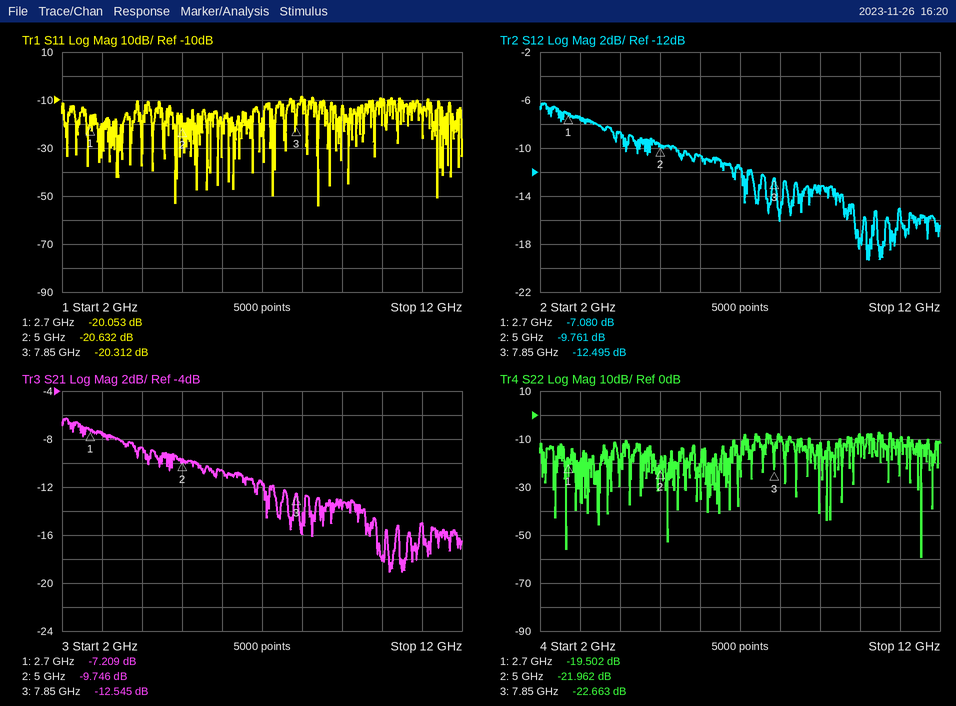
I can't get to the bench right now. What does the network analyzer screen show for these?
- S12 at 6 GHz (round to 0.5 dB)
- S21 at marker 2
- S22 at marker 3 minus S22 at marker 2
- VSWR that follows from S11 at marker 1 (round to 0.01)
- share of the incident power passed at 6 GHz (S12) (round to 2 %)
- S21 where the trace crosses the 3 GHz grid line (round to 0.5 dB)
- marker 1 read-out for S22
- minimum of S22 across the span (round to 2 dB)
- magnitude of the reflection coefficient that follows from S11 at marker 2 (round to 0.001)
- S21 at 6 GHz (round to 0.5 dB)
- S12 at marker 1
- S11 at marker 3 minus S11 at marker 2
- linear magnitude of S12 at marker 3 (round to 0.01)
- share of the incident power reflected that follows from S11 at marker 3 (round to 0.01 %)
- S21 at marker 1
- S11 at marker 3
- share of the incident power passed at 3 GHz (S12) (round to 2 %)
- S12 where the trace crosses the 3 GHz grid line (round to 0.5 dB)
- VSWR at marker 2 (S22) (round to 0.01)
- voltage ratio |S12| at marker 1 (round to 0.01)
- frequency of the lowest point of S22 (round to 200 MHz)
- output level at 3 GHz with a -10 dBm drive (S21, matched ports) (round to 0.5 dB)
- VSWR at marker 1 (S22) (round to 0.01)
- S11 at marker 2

-10.5 dB
-9.746 dB
-0.701 dB
1.22
8 %
-7.5 dB
-19.502 dB
-60 dB
0.093
-10.5 dB
-7.080 dB
0.320 dB
0.24
0.93 %
-7.209 dB
-20.312 dB
18 %
-7.5 dB
1.17
0.44
11.6 GHz
-17.5 dBm
1.24
-20.632 dB
